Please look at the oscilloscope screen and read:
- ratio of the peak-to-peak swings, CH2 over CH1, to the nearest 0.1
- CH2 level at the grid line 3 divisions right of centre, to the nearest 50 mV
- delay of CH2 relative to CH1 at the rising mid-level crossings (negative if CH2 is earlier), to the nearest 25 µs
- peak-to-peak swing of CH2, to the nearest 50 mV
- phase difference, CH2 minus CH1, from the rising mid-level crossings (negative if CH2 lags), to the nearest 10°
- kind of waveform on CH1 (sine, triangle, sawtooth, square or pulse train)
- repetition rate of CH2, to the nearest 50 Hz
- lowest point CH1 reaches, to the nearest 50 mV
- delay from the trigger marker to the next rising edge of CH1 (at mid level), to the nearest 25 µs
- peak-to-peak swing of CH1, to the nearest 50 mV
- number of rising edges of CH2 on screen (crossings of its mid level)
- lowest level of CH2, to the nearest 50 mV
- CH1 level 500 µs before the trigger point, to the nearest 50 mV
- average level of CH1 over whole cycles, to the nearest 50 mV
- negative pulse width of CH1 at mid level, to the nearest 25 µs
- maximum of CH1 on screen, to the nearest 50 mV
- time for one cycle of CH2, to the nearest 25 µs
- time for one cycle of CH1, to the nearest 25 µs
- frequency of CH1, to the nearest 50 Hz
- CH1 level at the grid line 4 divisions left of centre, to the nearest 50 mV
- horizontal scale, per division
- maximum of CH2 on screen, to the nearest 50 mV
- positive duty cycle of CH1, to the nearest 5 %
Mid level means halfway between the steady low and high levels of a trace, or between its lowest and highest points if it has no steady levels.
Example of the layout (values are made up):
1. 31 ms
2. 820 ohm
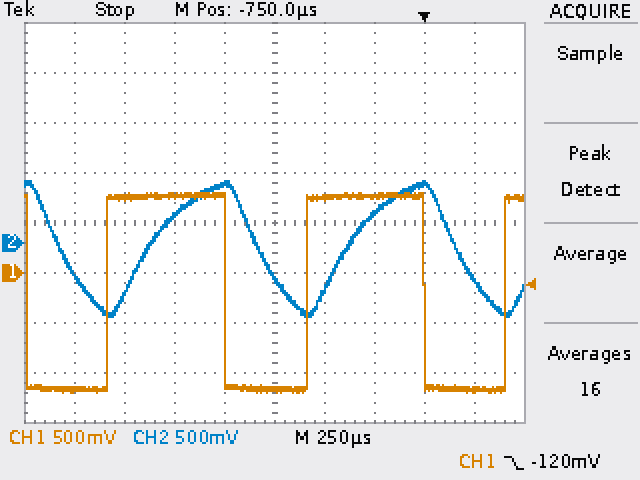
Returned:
1. 0.7
2. 600 mV
3. +200 µs
4. 1.35 V
5. -70°
6. pulse train
7. 1.00 kHz
8. -1.20 V
9. 400 µs
10. 2.00 V
11. 2
12. -750 mV
13. 750 mV
14. 0 mV
15. 400 µs
16. 800 mV
17. 1.000 ms
18. 1.000 ms
19. 1.00 kHz
20. -1.15 V
21. 250 µs
22. 600 mV
23. 60 %
